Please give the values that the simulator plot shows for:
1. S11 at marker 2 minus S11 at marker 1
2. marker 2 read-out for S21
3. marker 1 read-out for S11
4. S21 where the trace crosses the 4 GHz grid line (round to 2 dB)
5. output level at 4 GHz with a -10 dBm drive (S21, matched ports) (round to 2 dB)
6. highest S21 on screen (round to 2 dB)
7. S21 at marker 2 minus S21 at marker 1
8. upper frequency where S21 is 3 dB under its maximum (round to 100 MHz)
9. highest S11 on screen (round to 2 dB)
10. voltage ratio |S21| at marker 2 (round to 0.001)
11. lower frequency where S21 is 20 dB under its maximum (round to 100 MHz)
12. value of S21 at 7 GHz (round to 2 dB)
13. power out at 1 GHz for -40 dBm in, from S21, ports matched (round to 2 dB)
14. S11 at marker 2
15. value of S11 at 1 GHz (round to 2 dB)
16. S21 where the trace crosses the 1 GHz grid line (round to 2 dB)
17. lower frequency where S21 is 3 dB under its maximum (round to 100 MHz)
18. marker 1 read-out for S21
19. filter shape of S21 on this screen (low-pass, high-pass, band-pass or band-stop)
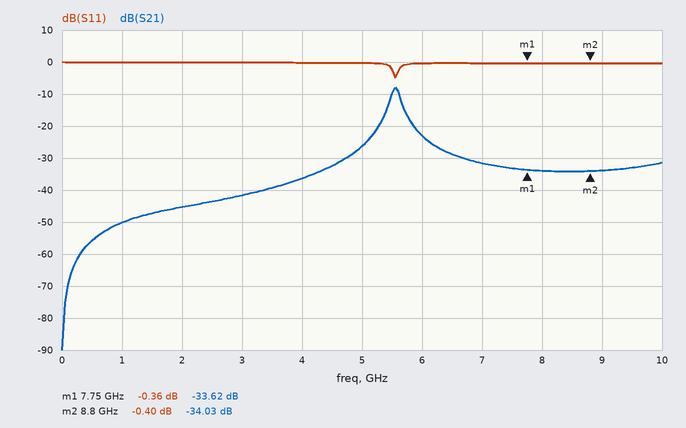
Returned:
-0.04 dB
-34.03 dB
-0.36 dB
-36 dB
-46 dBm
-8 dB
-0.41 dB
5.6 GHz
0 dB
0.020
4.9 GHz
-32 dB
-90 dBm
-0.40 dB
0 dB
-50 dB
5.5 GHz
-33.62 dB
band-pass
